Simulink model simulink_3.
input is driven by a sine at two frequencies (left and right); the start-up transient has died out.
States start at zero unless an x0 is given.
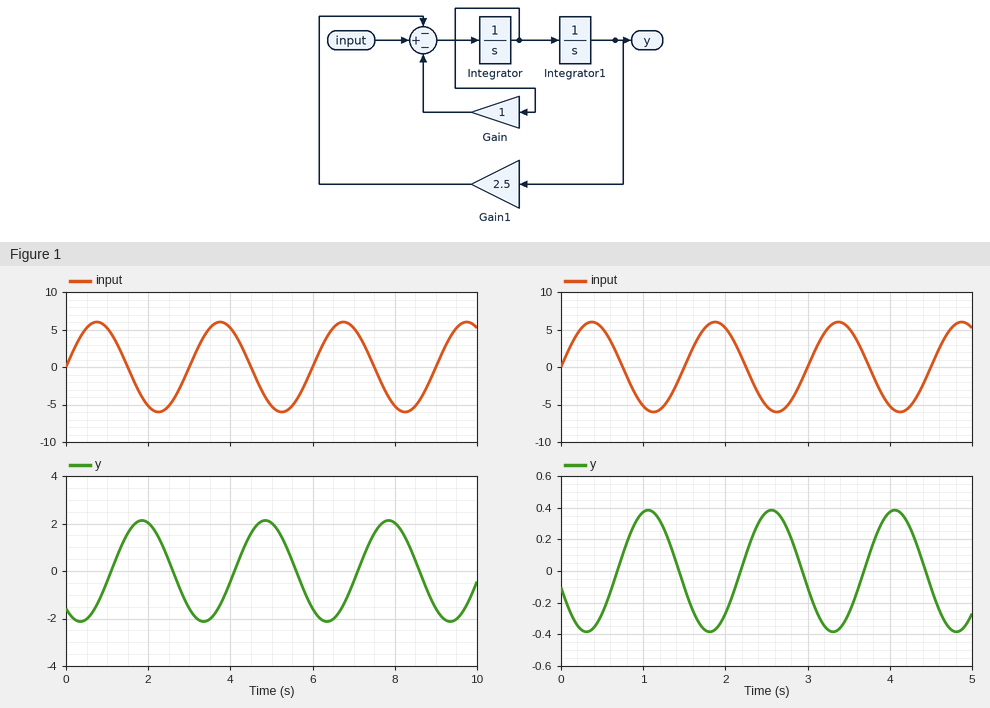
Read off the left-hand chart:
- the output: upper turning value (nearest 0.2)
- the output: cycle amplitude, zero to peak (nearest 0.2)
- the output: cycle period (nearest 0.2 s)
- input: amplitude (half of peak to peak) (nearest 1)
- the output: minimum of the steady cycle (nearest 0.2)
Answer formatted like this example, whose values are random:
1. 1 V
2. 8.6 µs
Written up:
1. 2.2
2. 2.2
3. 3.0 s
4. 6
5. -2.2
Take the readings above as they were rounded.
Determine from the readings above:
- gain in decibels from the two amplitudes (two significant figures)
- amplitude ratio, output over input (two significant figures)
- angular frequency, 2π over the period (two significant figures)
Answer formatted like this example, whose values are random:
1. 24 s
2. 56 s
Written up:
1. -8.7 dB
2. 0.37
3. 2.1 rad/s
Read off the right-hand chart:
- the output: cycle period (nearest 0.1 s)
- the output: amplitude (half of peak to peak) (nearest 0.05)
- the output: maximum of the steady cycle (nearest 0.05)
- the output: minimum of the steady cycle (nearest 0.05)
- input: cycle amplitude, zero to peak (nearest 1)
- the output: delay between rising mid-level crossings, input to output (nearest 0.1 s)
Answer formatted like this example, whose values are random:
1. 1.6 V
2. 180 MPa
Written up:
1. 1.5 s
2. 0.40
3. 0.40
4. -0.40
5. 6
6. 0.7 s
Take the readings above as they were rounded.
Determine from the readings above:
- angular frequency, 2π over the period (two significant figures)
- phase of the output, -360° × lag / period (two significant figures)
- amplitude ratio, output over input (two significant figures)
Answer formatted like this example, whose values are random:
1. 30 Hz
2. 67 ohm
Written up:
1. 4.2 rad/s
2. -170°
3. 0.067
